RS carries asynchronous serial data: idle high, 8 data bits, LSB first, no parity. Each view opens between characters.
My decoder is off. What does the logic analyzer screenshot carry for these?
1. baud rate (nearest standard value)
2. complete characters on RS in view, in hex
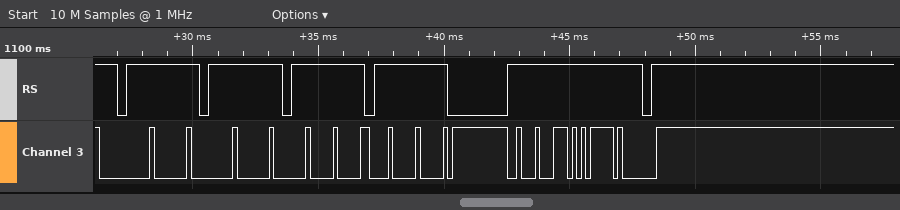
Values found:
2400 baud
7F, 7F, E0, FF
